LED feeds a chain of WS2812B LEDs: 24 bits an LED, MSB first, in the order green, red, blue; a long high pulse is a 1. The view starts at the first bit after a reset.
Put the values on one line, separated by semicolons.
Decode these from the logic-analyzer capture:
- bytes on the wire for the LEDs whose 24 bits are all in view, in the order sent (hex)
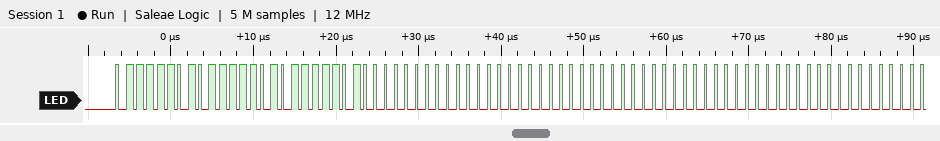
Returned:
7D 7D 7D 00 00 00 00 00 00
